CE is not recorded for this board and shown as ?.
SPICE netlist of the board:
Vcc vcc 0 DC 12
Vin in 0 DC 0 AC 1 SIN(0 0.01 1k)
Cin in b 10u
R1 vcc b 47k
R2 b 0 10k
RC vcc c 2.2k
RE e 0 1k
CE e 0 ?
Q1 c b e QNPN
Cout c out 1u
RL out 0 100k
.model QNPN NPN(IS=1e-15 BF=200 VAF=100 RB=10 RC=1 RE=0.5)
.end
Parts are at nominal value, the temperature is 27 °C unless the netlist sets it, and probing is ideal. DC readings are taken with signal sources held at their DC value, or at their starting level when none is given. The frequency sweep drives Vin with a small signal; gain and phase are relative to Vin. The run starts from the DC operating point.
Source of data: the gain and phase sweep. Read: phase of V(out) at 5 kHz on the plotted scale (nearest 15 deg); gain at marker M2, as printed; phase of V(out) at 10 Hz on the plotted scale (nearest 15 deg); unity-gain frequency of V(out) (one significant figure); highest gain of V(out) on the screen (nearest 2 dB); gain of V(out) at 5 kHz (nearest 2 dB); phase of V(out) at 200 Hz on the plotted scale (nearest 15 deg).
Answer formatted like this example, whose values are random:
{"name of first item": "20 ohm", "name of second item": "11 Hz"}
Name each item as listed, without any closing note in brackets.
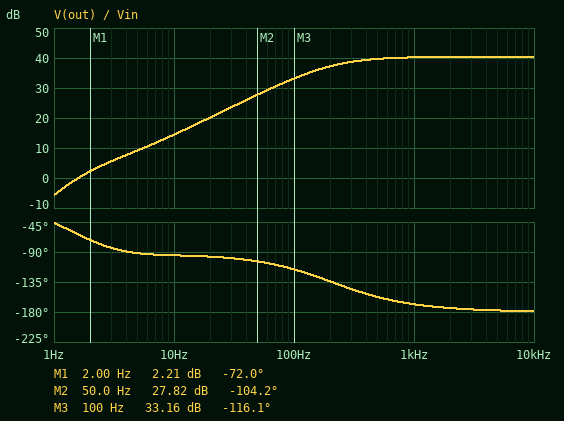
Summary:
{"phase of V(out) at 5 kHz on the plotted scale": "-180 deg", "gain at marker M2, as printed": "27.82 dB", "phase of V(out) at 10 Hz on the plotted scale": "-90 deg", "unity-gain frequency of V(out)": "2 Hz", "highest gain of V(out) on the screen": "40 dB", "gain of V(out) at 5 kHz": "40 dB", "phase of V(out) at 200 Hz on the plotted scale": "-135 deg"}
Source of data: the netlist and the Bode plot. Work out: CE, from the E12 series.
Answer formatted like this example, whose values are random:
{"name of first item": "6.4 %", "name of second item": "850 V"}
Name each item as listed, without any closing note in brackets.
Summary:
{"CE, from the E12 series": "39 µF"}
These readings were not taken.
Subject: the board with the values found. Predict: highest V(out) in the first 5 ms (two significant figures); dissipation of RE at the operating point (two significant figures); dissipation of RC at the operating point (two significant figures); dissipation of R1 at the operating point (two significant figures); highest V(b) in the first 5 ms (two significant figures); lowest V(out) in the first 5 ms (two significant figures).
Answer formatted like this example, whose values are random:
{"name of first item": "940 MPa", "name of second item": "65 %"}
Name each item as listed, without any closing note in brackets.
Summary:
{"highest V(out) in the first 5 ms": "960 mV", "dissipation of RE at the operating point": "1.8 mW", "dissipation of RC at the operating point": "3.9 mW", "dissipation of R1 at the operating point": "2.1 mW", "highest V(b) in the first 5 ms": "2.1 V", "lowest V(out) in the first 5 ms": "-1.1 V"}
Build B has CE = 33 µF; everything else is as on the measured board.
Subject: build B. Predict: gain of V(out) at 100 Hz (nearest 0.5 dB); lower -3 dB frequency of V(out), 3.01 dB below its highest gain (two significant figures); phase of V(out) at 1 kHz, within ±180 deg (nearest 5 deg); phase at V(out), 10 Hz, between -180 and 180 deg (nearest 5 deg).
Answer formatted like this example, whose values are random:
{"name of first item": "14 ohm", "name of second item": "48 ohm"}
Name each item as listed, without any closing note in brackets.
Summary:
{"gain of V(out) at 100 Hz": "32.0 dB", "lower -3 dB frequency of V(out), 3.01 dB below its highest gain": "240 Hz", "phase of V(out) at 1 kHz, within ±180 deg": "-165 deg", "phase at V(out), 10 Hz, between -180 and 180 deg": "-100 deg"}
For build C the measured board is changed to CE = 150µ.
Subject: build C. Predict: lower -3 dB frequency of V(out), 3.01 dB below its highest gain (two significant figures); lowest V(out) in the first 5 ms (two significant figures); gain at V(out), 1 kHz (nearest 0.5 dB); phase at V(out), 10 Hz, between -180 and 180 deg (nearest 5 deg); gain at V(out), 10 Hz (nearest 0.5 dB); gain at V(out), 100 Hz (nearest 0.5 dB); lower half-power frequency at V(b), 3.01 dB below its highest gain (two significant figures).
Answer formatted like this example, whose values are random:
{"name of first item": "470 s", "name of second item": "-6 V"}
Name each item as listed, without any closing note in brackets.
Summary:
{"lower -3 dB frequency of V(out), 3.01 dB below its highest gain": "57 Hz", "lowest V(out) in the first 5 ms": "-1.2 V", "gain at V(out), 1 kHz": "40.5 dB", "phase at V(out), 10 Hz, between -180 and 180 deg": "-85 deg", "gain at V(out), 10 Hz": "25.0 dB", "gain at V(out), 100 Hz": "39.0 dB", "lower half-power frequency at V(b), 3.01 dB below its highest gain": "2.2 Hz"}
